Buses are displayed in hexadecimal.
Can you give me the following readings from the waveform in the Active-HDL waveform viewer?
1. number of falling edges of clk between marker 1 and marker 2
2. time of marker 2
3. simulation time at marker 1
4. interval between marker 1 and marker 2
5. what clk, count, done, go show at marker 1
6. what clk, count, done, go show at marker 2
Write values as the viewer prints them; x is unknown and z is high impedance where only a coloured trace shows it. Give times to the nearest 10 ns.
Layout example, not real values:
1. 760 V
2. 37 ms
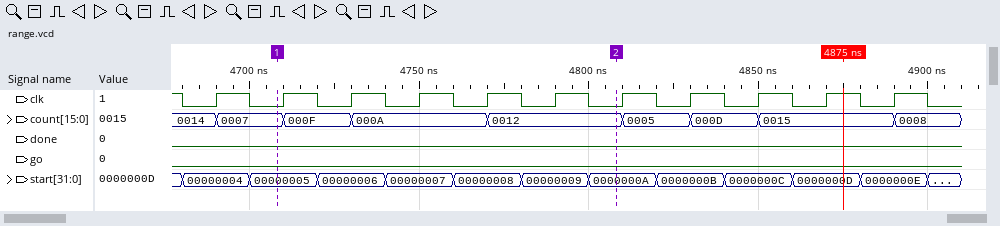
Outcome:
1. 5
2. 4810 ns
3. 4710 ns
4. 100 ns
5. clk=0, count=0007, done=0, go=0
6. clk=0, count=0012, done=0, go=0
